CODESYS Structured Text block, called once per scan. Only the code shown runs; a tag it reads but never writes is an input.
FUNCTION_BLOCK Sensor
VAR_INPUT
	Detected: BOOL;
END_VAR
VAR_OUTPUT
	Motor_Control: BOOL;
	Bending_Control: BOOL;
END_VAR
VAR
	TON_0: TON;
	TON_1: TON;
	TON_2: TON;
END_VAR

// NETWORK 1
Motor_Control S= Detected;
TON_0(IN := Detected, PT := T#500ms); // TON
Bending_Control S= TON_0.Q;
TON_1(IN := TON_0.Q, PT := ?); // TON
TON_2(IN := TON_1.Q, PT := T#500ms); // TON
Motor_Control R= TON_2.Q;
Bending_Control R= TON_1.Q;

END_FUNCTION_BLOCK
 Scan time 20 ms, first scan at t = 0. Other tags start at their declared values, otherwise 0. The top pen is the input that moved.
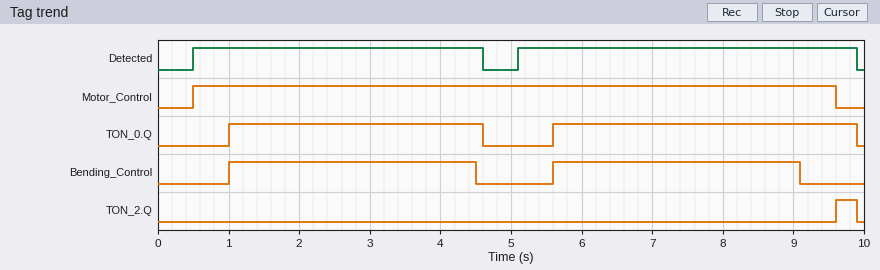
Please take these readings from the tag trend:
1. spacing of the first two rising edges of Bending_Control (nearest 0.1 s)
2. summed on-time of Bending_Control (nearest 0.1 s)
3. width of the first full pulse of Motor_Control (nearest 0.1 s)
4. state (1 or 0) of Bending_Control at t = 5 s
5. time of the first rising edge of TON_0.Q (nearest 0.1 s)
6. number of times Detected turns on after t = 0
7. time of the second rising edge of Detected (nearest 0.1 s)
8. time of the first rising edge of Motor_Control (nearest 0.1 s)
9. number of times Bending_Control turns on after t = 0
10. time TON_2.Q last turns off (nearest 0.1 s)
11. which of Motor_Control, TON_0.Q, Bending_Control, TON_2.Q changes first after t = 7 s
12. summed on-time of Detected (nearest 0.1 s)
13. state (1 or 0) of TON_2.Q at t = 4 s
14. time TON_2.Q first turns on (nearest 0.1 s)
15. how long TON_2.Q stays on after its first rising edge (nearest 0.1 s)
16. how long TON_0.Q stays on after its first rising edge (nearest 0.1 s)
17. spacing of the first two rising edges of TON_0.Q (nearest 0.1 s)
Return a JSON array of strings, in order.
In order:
["4.6 s", "7.0 s", "9.1 s", "0", "1.0 s", "2", "5.1 s", "0.5 s", "2", "9.9 s", "Bending_Control", "8.9 s", "0", "9.6 s", "0.3 s", "3.6 s", "4.6 s"]
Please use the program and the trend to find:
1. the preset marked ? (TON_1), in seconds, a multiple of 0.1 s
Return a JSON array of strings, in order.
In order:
["3.5 s"]
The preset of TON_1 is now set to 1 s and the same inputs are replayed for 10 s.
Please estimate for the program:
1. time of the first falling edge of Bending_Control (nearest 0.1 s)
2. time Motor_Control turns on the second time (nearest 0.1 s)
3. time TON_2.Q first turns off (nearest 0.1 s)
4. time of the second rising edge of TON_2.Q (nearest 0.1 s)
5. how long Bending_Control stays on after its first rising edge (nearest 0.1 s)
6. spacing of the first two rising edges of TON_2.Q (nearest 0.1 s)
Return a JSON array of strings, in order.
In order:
["2.0 s", "5.1 s", "4.6 s", "7.1 s", "1.0 s", "4.6 s"]
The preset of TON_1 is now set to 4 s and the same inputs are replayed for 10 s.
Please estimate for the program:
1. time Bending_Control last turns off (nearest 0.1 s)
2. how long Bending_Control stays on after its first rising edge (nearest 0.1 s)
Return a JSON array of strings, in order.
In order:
["9.6 s", "8.6 s"]
